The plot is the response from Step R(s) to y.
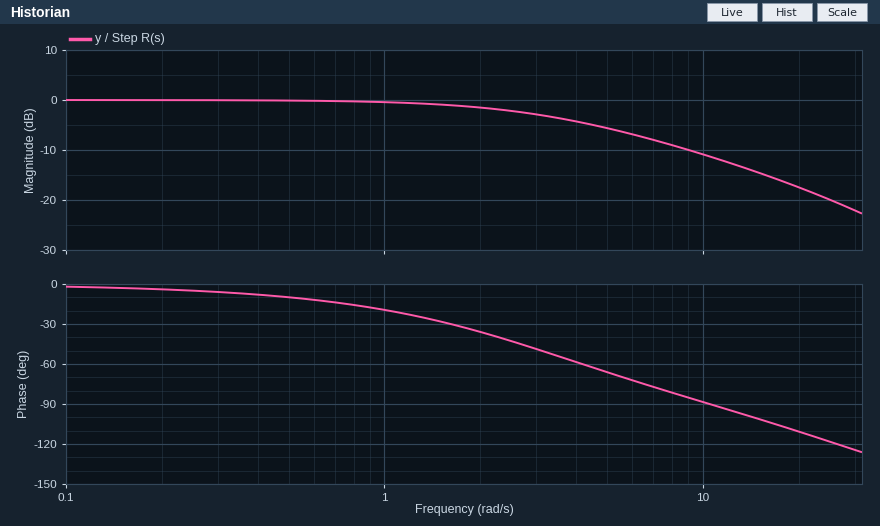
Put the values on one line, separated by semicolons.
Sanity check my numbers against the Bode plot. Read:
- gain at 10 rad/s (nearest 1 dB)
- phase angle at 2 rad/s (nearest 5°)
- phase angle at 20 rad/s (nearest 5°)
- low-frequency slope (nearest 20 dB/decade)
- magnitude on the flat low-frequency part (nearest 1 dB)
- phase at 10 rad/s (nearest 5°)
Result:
-11 dB; -35°; -110°; 0 dB/decade; 0 dB; -90°
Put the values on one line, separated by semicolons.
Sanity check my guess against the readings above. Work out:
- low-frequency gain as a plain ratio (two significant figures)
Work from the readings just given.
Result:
1.0
